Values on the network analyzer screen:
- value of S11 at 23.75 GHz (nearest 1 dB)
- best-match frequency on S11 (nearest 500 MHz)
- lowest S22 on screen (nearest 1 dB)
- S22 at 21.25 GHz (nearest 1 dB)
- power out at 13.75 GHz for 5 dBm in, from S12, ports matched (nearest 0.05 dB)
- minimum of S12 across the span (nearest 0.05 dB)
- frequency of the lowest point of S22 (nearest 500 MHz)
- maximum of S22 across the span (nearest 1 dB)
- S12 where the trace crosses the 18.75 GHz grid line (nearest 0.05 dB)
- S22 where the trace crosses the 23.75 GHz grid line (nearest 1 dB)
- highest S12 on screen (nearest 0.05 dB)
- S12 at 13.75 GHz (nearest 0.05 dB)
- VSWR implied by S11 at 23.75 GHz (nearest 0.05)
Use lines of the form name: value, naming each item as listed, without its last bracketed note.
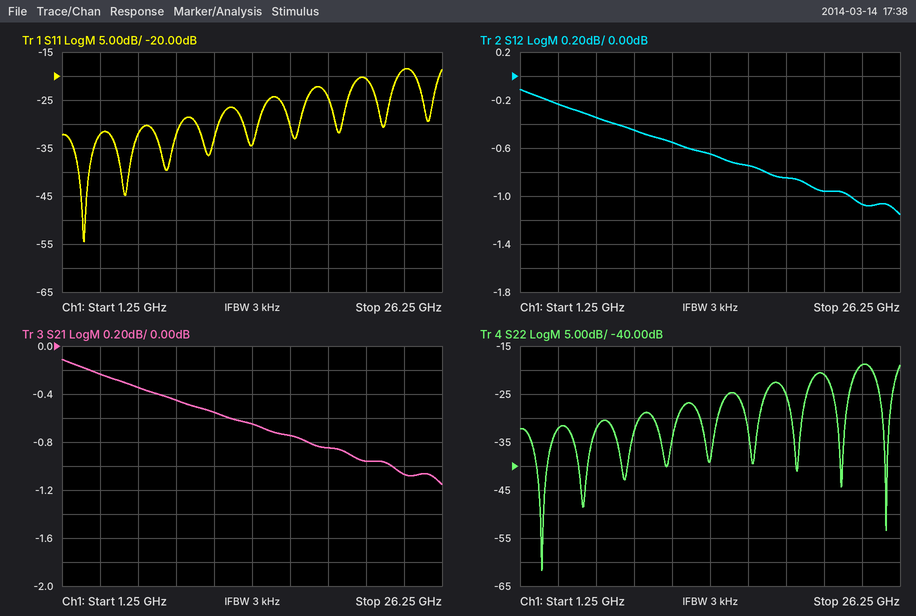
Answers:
value of S11 at 23.75 GHz: -19 dB
best-match frequency on S11: 2.5 GHz
lowest S22 on screen: -62 dB
S22 at 21.25 GHz: -21 dB
power out at 13.75 GHz for 5 dBm in, from S12, ports matched: 4.35 dBm
minimum of S12 across the span: -1.15 dB
frequency of the lowest point of S22: 2.5 GHz
maximum of S22 across the span: -19 dB
S12 where the trace crosses the 18.75 GHz grid line: -0.85 dB
S22 where the trace crosses the 23.75 GHz grid line: -19 dB
highest S12 on screen: -0.10 dB
S12 at 13.75 GHz: -0.65 dB
VSWR implied by S11 at 23.75 GHz: 1.25
